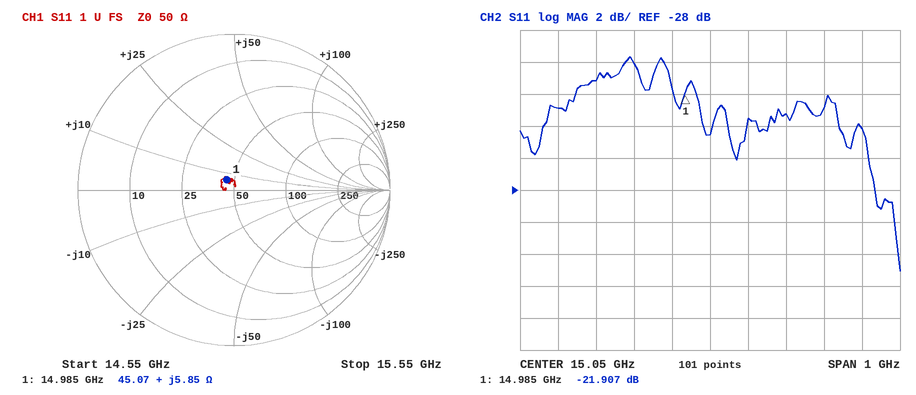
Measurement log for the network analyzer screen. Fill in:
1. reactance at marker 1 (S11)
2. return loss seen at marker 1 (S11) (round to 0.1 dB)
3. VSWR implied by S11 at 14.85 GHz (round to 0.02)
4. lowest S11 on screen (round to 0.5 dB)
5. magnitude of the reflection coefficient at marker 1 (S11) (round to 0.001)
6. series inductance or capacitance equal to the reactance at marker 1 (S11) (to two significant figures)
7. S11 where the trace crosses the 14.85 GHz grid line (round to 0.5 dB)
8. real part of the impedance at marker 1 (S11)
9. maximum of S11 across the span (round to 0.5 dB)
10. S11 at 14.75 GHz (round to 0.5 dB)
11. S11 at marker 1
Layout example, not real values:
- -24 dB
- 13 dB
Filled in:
- +5.85 Ω
- 21.9 dB
- 1.22
- -33.0 dB
- 0.080
- 62 pH
- -20.0 dB
- 45.07 Ω
- -19.5 dB
- -21.0 dB
- -21.907 dB
